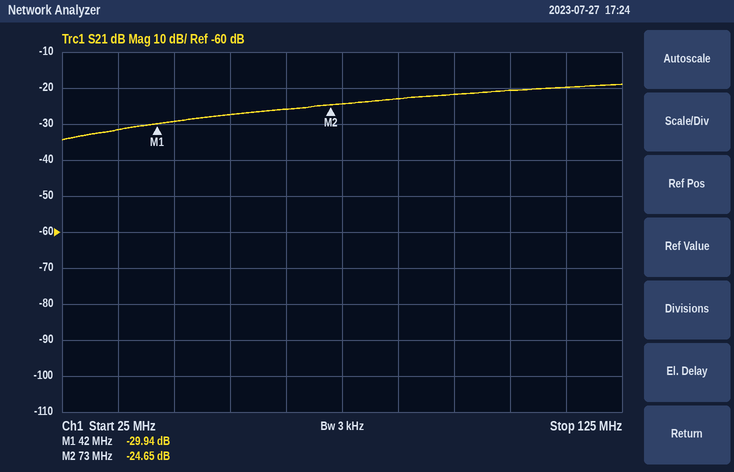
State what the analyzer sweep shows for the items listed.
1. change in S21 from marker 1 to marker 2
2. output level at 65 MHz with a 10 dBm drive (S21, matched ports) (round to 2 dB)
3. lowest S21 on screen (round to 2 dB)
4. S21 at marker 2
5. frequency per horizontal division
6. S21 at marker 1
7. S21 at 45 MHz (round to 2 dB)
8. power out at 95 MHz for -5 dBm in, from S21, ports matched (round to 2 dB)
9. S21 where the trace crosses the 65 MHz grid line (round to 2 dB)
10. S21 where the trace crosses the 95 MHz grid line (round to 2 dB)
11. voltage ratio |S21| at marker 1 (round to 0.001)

5.29 dB
-16 dBm
-34 dB
-24.65 dB
10 MHz
-29.94 dB
-30 dB
-26 dBm
-26 dB
-22 dB
0.032
